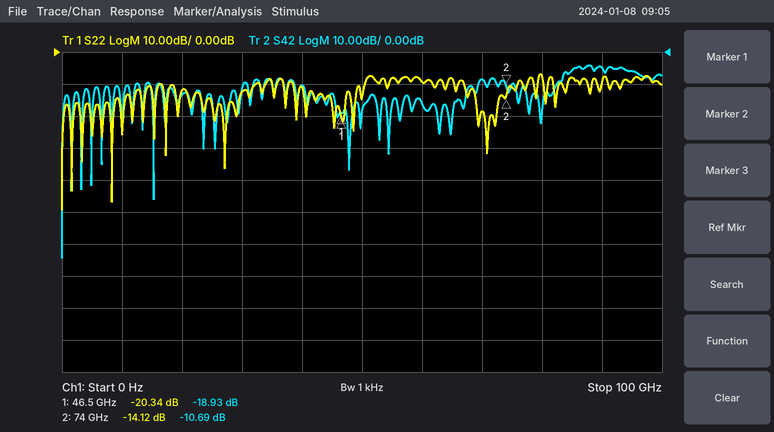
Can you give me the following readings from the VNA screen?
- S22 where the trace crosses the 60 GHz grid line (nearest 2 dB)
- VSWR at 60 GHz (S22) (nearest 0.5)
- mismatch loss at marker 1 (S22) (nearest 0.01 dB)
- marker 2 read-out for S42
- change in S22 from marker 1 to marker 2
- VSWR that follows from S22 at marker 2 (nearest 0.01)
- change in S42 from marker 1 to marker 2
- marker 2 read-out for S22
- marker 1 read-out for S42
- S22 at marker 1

-10 dB
2.0
0.04 dB
-10.69 dB
6.22 dB
1.49
8.24 dB
-14.12 dB
-18.93 dB
-20.34 dB
